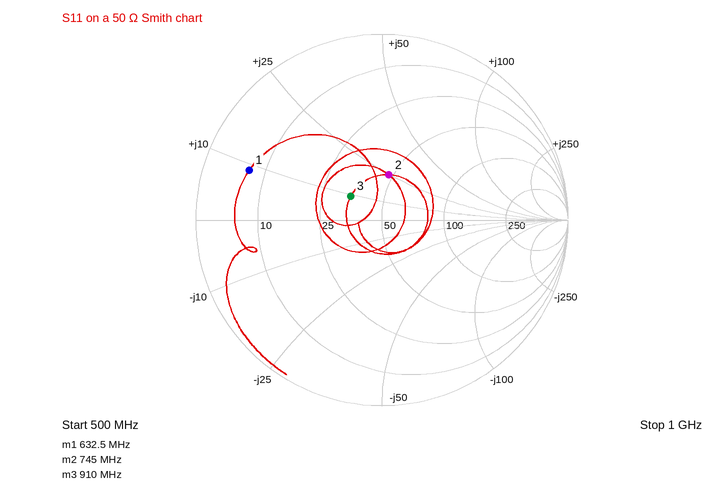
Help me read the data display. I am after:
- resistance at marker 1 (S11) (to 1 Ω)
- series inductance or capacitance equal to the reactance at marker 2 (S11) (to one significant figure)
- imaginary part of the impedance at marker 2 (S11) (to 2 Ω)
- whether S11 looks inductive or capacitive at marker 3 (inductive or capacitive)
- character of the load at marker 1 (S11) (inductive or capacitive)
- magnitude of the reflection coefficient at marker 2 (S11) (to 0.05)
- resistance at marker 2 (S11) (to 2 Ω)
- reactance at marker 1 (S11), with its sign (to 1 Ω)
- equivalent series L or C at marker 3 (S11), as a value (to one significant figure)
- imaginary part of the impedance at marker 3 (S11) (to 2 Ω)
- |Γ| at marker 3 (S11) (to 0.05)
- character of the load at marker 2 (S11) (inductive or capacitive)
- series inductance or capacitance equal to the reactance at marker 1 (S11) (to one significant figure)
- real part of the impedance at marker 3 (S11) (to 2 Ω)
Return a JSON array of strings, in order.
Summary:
["7 Ω", "5 nH", "+24 Ω", "inductive", "inductive", "0.25", "48 Ω", "+9 Ω", "2 nH", "+10 Ω", "0.20", "inductive", "2 nH", "34 Ω"]
